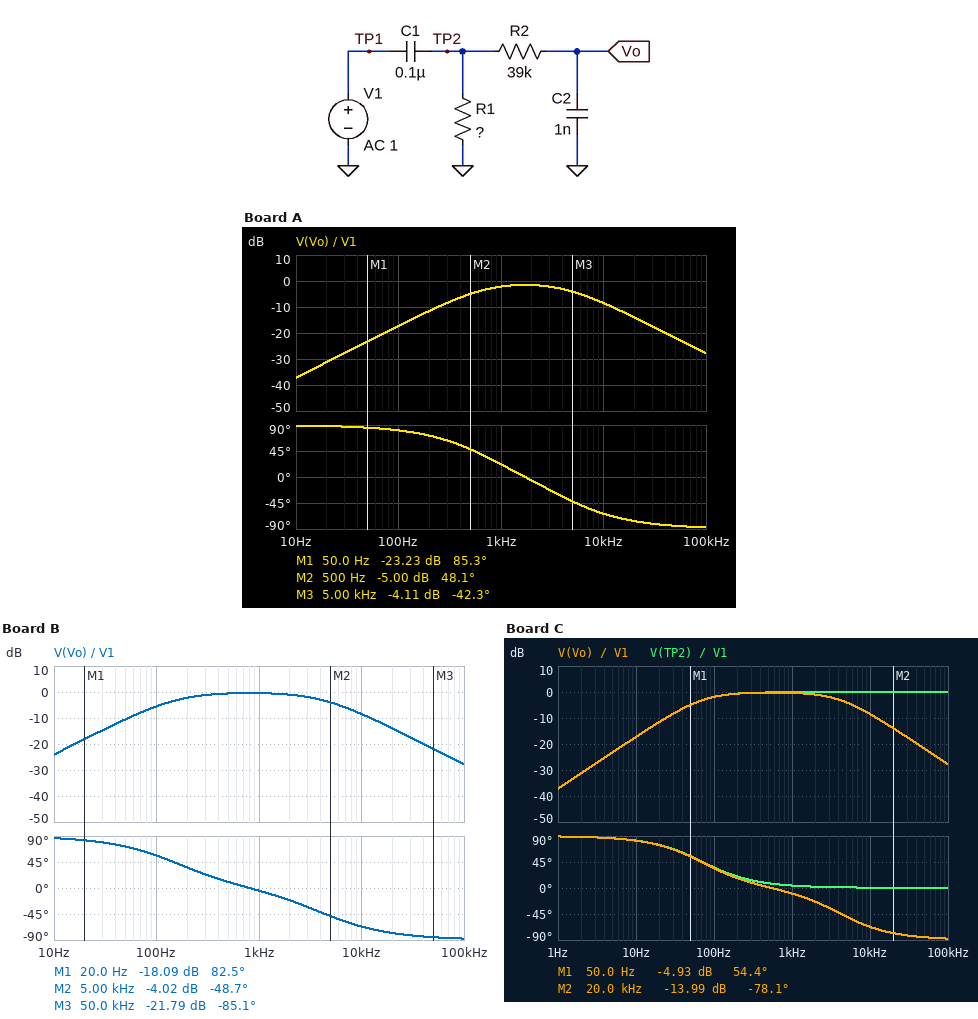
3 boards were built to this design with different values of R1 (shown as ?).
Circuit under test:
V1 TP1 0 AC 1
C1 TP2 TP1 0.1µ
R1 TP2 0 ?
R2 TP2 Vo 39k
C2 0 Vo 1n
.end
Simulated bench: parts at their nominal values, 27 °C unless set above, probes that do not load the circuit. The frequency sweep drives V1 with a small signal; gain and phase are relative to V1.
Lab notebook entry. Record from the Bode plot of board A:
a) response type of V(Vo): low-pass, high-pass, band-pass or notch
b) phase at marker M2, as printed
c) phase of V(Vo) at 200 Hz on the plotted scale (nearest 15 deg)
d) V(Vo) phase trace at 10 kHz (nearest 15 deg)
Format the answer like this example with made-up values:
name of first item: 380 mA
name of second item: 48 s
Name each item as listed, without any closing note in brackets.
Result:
response type of V(Vo): low-pass, high-pass, band-pass or notch: band-pass
phase at marker M2, as printed: 48.1 deg
phase of V(Vo) at 200 Hz on the plotted scale: 75 deg
V(Vo) phase trace at 10 kHz: -60 deg
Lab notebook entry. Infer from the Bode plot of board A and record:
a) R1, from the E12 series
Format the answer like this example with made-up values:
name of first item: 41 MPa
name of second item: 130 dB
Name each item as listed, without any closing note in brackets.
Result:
R1, from the E12 series: 2.2 kΩ
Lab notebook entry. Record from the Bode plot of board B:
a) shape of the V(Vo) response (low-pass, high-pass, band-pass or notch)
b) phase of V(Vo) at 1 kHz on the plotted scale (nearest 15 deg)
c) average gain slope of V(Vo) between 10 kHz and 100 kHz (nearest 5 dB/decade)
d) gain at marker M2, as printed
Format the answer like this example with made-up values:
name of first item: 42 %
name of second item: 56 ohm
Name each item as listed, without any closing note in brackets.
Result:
shape of the V(Vo) response: band-pass
phase of V(Vo) at 1 kHz on the plotted scale: 0 deg
average gain slope of V(Vo) between 10 kHz and 100 kHz: -20 dB/decade
gain at marker M2, as printed: -4.02 dB
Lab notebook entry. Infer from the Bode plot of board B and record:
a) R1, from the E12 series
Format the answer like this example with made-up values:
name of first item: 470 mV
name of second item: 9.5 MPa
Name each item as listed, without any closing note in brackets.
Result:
R1, from the E12 series: 10 kΩ
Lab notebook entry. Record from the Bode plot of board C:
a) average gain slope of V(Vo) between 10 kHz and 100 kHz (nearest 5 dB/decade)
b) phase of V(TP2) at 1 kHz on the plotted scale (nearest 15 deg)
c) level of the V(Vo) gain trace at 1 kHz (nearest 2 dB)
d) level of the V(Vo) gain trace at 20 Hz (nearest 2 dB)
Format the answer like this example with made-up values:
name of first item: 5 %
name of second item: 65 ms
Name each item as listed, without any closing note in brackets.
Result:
average gain slope of V(Vo) between 10 kHz and 100 kHz: -20 dB/decade
phase of V(TP2) at 1 kHz on the plotted scale: 0 deg
level of the V(Vo) gain trace at 1 kHz: 0 dB
level of the V(Vo) gain trace at 20 Hz: -12 dB
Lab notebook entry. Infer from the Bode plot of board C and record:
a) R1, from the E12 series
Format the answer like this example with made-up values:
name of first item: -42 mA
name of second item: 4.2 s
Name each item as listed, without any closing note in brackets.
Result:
R1, from the E12 series: 22 kΩ
